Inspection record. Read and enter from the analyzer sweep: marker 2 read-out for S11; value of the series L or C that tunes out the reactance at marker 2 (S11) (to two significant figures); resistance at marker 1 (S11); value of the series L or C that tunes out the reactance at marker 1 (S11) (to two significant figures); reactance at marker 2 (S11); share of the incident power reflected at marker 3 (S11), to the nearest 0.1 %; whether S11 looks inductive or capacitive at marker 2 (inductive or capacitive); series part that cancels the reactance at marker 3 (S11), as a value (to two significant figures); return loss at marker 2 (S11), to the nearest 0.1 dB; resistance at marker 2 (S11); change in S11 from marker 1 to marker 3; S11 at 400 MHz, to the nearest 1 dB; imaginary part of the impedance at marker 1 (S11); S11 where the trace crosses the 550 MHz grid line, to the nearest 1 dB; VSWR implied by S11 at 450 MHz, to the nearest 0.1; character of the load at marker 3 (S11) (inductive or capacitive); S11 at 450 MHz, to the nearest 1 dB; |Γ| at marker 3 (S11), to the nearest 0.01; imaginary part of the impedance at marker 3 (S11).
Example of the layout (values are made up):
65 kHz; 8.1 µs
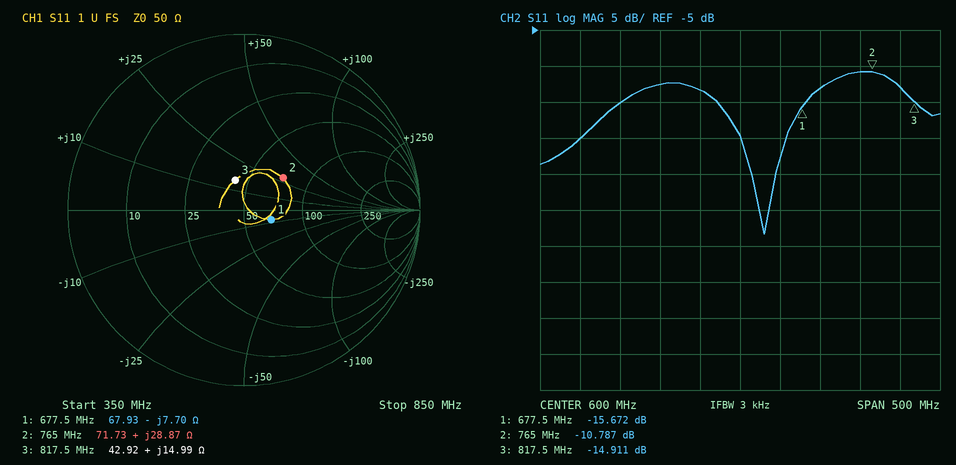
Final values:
-10.787 dB; 7.2 pF; 67.93 Ω; 1.8 nH; +28.87 Ω; 3.2 %; inductive; 13 pF; 10.8 dB; 71.73 Ω; 0.761 dB; -20 dB; -7.70 Ω; -13 dB; 1.4; inductive; -15 dB; 0.18; +14.99 Ω
